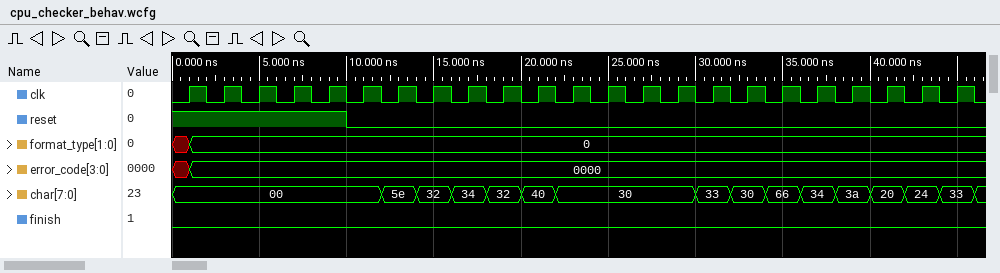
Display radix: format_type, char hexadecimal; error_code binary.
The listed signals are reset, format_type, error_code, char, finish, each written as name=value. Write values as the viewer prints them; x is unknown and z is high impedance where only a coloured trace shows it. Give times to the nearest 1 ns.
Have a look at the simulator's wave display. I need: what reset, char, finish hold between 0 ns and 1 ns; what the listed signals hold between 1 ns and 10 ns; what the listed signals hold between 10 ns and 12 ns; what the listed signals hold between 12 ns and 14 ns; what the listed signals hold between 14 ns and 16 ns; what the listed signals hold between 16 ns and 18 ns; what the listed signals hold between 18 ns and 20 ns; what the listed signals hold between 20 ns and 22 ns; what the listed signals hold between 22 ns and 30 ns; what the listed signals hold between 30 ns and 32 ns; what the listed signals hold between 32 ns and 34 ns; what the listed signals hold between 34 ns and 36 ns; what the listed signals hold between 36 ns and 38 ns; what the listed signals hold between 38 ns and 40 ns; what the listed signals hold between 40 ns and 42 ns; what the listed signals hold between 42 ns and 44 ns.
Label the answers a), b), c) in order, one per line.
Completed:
a) reset=1, char=00, finish=0
b) reset=1, format_type=0, error_code=0000, char=00, finish=0
c) reset=0, format_type=0, error_code=0000, char=00, finish=0
d) reset=0, format_type=0, error_code=0000, char=5e, finish=0
e) reset=0, format_type=0, error_code=0000, char=32, finish=0
f) reset=0, format_type=0, error_code=0000, char=34, finish=0
g) reset=0, format_type=0, error_code=0000, char=32, finish=0
h) reset=0, format_type=0, error_code=0000, char=40, finish=0
i) reset=0, format_type=0, error_code=0000, char=30, finish=0
j) reset=0, format_type=0, error_code=0000, char=33, finish=0
k) reset=0, format_type=0, error_code=0000, char=30, finish=0
l) reset=0, format_type=0, error_code=0000, char=66, finish=0
m) reset=0, format_type=0, error_code=0000, char=34, finish=0
n) reset=0, format_type=0, error_code=0000, char=3a, finish=0
o) reset=0, format_type=0, error_code=0000, char=20, finish=0
p) reset=0, format_type=0, error_code=0000, char=24, finish=0
